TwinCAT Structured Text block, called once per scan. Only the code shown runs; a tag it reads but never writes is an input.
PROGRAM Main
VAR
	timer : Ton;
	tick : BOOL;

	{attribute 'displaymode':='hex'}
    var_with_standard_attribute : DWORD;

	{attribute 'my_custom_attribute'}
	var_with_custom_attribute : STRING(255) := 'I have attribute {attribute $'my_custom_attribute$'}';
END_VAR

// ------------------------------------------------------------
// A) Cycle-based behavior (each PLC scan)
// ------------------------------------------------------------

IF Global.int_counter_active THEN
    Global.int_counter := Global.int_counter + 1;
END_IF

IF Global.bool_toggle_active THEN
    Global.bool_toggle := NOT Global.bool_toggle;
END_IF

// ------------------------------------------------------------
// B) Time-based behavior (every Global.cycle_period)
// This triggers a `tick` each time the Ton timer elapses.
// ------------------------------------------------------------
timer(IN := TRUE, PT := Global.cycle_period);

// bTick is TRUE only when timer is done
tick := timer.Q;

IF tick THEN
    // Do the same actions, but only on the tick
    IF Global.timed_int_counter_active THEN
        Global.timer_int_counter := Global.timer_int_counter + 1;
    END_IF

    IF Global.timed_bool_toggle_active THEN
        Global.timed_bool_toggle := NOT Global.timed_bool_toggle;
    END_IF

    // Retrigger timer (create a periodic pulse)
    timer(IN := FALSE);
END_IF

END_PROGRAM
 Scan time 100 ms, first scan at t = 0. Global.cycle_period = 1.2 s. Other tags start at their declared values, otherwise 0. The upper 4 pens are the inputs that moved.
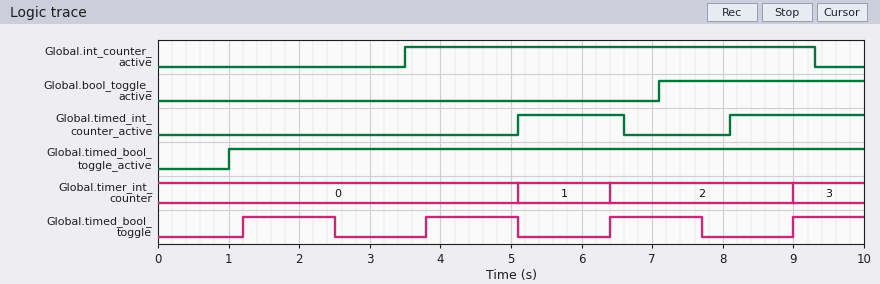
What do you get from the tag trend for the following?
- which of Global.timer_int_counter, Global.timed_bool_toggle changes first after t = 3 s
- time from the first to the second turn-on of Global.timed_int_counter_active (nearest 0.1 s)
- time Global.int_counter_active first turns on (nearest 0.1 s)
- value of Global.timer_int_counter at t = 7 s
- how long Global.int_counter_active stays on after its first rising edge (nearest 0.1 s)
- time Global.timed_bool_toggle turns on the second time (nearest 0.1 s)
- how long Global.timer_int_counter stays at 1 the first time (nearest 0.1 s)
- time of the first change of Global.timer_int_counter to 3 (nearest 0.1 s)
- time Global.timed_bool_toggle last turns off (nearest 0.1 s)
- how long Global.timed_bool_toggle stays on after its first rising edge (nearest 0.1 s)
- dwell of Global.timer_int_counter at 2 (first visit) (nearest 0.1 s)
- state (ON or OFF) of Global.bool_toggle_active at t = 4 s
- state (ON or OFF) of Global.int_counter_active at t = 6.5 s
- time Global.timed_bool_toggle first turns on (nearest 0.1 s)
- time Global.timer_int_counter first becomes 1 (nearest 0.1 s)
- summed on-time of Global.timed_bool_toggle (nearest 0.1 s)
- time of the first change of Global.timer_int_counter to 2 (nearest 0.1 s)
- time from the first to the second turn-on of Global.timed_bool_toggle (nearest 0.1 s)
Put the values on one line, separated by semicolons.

Global.timed_bool_toggle; 3.0 s; 3.5 s; 2; 5.8 s; 3.8 s; 1.3 s; 9.0 s; 7.7 s; 1.3 s; 2.6 s; OFF; ON; 1.2 s; 5.1 s; 4.9 s; 6.4 s; 2.6 s
